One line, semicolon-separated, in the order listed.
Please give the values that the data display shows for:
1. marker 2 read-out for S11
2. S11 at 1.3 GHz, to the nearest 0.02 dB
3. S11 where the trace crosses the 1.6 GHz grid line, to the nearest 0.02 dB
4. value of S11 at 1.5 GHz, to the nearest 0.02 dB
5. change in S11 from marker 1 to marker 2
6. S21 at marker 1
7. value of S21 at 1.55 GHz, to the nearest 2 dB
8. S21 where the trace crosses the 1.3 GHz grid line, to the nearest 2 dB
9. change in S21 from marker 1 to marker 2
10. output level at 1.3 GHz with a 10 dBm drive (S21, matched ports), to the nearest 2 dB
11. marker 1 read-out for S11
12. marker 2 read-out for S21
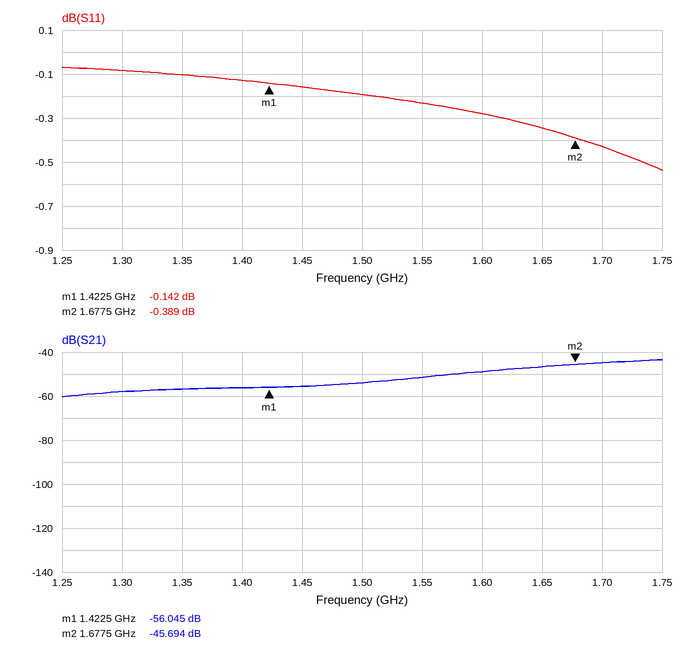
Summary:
-0.389 dB; -0.08 dB; -0.28 dB; -0.20 dB; -0.247 dB; -56.045 dB; -52 dB; -58 dB; 10.351 dB; -48 dBm; -0.142 dB; -45.694 dB
